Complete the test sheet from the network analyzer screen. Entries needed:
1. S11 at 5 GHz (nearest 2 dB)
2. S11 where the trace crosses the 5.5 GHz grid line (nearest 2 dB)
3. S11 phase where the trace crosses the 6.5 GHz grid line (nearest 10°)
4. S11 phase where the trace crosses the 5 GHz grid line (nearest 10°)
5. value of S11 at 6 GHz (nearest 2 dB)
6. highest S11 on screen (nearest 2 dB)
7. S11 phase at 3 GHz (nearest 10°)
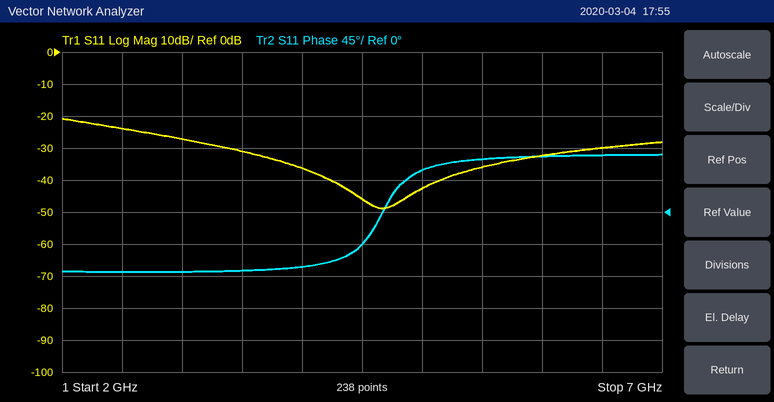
-42 dB
-36 dB
80°
60°
-32 dB
-20 dB
-80°
